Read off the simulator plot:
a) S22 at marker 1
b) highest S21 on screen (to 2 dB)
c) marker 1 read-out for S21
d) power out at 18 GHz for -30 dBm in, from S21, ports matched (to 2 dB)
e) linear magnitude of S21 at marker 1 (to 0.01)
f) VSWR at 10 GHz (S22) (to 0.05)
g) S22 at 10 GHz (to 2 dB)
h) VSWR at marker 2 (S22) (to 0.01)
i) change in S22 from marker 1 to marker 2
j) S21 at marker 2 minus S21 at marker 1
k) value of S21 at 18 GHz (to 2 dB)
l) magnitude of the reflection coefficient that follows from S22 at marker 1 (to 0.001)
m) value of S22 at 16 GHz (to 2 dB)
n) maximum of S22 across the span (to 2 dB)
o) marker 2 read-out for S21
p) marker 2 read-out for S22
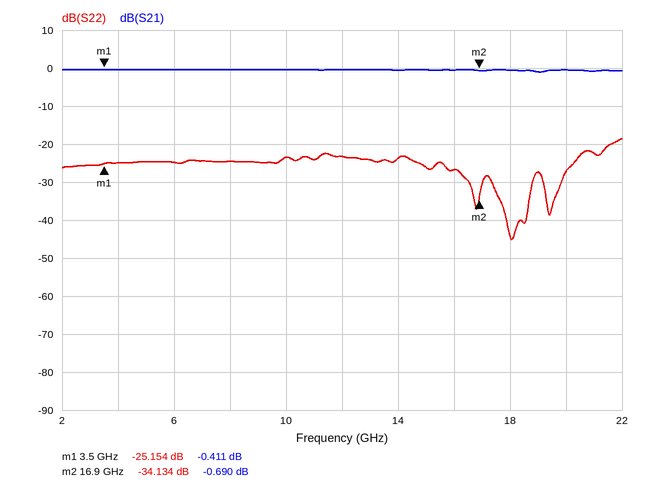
-25.154 dB
0 dB
-0.411 dB
-30 dBm
0.95
1.15
-24 dB
1.04
-8.980 dB
-0.279 dB
0 dB
0.055
-26 dB
-18 dB
-0.690 dB
-34.134 dB
